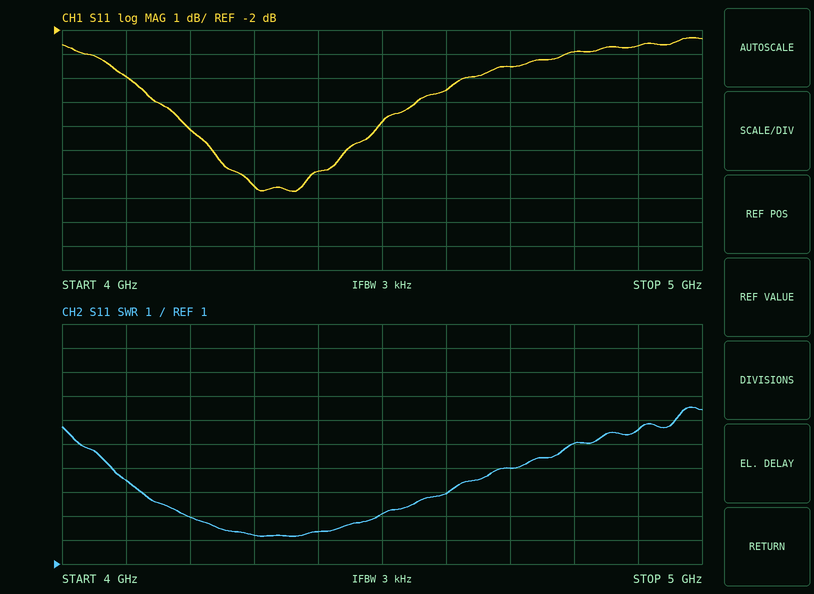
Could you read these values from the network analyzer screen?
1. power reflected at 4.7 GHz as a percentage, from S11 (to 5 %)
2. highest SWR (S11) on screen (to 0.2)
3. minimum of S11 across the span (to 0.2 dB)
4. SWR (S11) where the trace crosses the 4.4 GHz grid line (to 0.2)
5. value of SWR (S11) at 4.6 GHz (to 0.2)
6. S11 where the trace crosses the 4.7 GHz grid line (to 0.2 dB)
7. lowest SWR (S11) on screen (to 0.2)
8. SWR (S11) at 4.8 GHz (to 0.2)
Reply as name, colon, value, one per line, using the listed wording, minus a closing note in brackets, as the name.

power reflected at 4.7 GHz as a percentage, from S11: 45 %
highest SWR (S11) on screen: 7.6
minimum of S11 across the span: -8.8 dB
SWR (S11) where the trace crosses the 4.4 GHz grid line: 2.4
value of SWR (S11) at 4.6 GHz: 4.0
S11 where the trace crosses the 4.7 GHz grid line: -3.6 dB
lowest SWR (S11) on screen: 2.2
SWR (S11) at 4.8 GHz: 6.0
